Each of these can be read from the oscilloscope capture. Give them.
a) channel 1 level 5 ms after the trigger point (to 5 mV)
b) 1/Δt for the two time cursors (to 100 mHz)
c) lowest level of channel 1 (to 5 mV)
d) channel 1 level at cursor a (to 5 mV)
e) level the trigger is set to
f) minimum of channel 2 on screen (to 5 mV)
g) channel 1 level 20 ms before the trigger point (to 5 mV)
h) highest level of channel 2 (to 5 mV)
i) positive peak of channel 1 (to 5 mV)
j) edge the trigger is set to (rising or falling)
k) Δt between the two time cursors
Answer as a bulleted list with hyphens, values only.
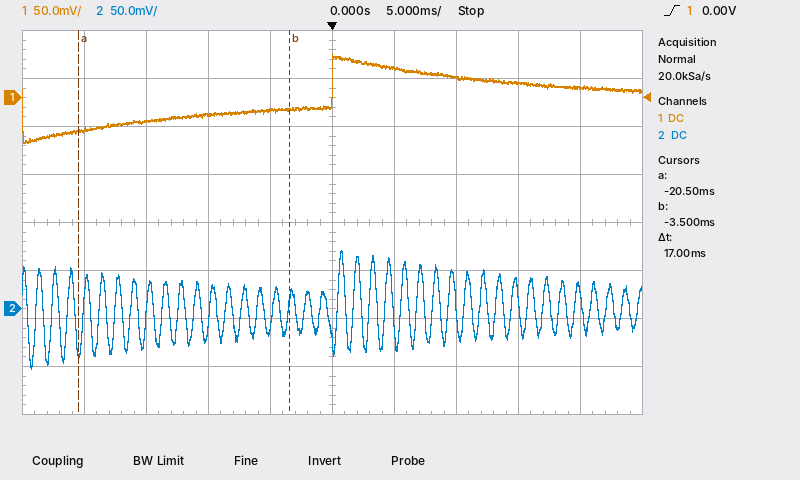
- 30 mV
- 58.8 Hz
- -45 mV
- -35 mV
- 0.00 V
- -60 mV
- -35 mV
- 60 mV
- 45 mV
- rising
- 17 ms
